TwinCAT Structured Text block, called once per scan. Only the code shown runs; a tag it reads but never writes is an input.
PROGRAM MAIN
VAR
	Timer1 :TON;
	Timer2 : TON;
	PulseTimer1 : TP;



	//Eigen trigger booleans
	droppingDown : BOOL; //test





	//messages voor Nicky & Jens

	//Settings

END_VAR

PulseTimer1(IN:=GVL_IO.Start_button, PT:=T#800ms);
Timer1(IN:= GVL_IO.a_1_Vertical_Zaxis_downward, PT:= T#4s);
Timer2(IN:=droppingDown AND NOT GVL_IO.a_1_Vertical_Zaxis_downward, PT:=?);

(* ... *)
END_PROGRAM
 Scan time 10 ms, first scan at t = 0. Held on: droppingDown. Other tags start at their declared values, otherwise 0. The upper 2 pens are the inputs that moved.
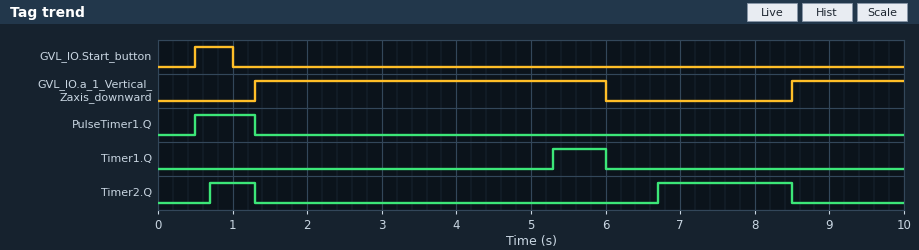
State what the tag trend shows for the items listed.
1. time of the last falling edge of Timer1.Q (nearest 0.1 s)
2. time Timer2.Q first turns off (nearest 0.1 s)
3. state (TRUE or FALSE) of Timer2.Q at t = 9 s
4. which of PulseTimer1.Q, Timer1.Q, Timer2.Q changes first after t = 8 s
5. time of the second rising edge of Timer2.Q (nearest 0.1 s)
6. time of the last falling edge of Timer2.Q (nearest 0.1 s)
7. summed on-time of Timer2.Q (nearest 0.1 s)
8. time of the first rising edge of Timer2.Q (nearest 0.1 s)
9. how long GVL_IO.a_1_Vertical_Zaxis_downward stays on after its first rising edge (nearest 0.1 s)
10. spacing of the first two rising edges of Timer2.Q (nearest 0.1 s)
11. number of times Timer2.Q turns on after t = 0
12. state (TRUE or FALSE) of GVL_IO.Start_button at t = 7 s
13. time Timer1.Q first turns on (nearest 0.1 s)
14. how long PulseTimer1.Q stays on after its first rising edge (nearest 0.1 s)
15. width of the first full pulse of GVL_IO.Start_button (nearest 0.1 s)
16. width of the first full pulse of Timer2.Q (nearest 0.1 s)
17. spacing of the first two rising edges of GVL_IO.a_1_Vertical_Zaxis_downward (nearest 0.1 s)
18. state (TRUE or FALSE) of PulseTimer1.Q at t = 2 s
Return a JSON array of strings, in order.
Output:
["6.0 s", "1.3 s", "FALSE", "Timer2.Q", "6.7 s", "8.5 s", "2.4 s", "0.7 s", "4.7 s", "6.0 s", "2", "FALSE", "5.3 s", "0.8 s", "0.5 s", "0.6 s", "7.2 s", "FALSE"]
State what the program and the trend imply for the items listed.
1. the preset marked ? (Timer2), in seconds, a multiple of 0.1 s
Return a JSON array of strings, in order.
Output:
["0.7 s"]
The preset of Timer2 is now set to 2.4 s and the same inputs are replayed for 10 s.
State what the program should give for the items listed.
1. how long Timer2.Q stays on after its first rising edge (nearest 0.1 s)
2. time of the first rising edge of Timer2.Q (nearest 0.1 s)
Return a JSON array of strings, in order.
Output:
["0.1 s", "8.4 s"]
